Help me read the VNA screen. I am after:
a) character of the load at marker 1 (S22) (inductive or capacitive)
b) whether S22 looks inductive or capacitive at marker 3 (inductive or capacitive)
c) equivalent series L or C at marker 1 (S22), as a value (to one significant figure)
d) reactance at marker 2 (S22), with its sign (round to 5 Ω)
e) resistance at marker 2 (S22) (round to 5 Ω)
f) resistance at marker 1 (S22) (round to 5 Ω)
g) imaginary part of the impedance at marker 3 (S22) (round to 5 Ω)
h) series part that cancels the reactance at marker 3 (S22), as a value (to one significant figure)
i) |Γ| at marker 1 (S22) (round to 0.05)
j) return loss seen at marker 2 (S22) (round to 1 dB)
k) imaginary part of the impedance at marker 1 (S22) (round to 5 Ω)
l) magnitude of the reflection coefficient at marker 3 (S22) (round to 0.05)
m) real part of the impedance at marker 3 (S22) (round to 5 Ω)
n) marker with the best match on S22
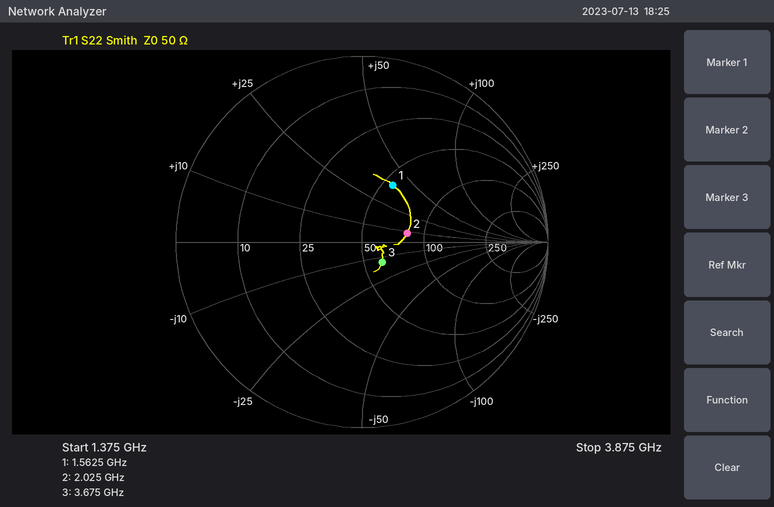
inductive
capacitive
4 nH
+10 Ω
80 Ω
55 Ω
-15 Ω
600 pH
0.35
12 dB
+40 Ω
0.15
60 Ω
marker 3
